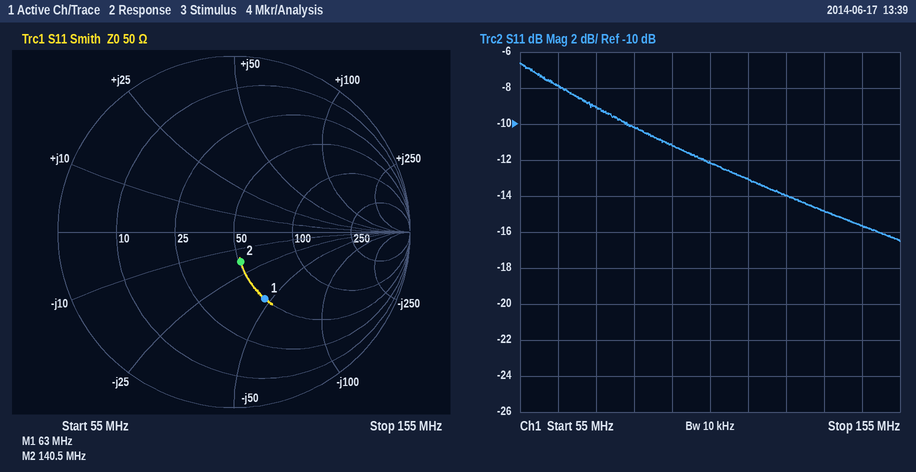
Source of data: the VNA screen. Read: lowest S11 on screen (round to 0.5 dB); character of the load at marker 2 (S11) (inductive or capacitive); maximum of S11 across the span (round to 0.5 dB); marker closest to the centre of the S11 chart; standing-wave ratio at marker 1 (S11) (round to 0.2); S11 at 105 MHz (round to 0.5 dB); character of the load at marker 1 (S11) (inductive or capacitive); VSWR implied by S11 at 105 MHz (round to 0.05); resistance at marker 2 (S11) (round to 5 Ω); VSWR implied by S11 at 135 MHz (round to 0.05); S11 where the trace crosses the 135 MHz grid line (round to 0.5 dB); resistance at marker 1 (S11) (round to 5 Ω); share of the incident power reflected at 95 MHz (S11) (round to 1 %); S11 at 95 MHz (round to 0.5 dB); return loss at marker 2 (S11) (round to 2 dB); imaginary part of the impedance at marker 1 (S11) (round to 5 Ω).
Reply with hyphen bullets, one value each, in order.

- -16.5 dB
- capacitive
- -6.5 dB
- marker 2
- 2.4
- -12.0 dB
- capacitive
- 1.65
- 50 Ω
- 1.45
- -15.0 dB
- 50 Ω
- 8 %
- -11.0 dB
- 16 dB
- -45 Ω
